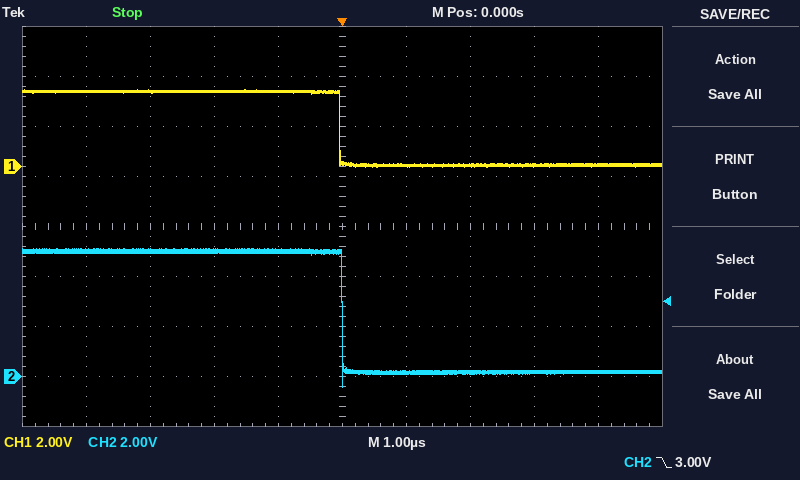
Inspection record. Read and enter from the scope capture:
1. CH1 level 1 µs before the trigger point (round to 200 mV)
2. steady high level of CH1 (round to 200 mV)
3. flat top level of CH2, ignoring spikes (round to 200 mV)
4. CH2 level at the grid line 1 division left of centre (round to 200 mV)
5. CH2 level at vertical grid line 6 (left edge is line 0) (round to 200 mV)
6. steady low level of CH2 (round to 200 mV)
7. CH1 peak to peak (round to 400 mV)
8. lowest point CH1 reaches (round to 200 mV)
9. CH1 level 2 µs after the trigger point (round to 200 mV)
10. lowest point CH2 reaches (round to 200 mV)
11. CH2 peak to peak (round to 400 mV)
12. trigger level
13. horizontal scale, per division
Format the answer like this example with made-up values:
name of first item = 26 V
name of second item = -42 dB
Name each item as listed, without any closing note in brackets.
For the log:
CH1 level 1 µs before the trigger point = 3.0 V
steady high level of CH1 = 3.0 V
flat top level of CH2, ignoring spikes = 5.0 V
CH2 level at the grid line 1 division left of centre = 5.0 V
CH2 level at vertical grid line 6 (left edge is line 0) = 200 mV
steady low level of CH2 = 200 mV
CH1 peak to peak = 3.2 V
lowest point CH1 reaches = 0.0 V
CH1 level 2 µs after the trigger point = 0.0 V
lowest point CH2 reaches = -400 mV
CH2 peak to peak = 5.6 V
trigger level = 3.00 V
horizontal scale, per division = 1 µs
